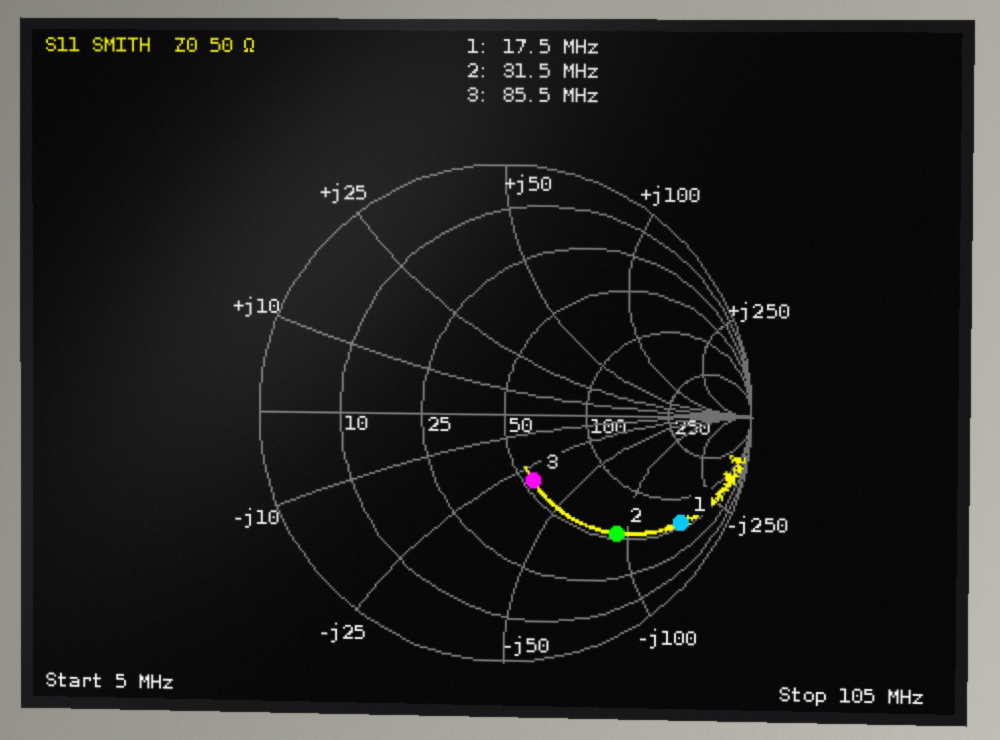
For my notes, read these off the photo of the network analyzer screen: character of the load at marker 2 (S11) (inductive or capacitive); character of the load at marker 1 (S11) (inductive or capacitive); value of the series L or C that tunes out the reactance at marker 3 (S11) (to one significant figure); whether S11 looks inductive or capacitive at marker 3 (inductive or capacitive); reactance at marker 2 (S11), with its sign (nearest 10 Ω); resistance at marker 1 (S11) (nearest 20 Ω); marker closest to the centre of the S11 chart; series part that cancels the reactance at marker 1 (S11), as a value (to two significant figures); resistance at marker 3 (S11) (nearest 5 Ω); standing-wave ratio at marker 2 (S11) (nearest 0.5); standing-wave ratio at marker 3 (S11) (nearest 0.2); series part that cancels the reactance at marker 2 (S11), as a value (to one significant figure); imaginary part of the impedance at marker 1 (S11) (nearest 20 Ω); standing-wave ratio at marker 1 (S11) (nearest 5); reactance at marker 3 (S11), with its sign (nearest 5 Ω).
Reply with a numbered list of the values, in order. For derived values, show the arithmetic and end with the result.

1. capacitive
2. capacitive
3. L = 30 Ω/(2π × 85.5 MHz) ≈ 55.8 nH, so 60 nH to one significant figure
4. capacitive
5. -90 Ω
6. 60 Ω
7. marker 3
8. L = 160 Ω/(2π × 17.5 MHz) ≈ 1.5 µH
9. 55 Ω
10. 5.0
11. 1.8
12. L = 90 Ω/(2π × 31.5 MHz) ≈ 455 nH, so 500 nH to one significant figure
13. -160 Ω
14. 10
15. -30 Ω
